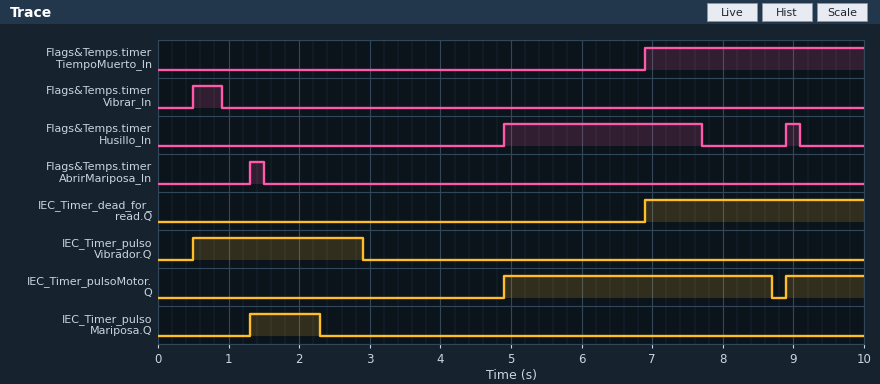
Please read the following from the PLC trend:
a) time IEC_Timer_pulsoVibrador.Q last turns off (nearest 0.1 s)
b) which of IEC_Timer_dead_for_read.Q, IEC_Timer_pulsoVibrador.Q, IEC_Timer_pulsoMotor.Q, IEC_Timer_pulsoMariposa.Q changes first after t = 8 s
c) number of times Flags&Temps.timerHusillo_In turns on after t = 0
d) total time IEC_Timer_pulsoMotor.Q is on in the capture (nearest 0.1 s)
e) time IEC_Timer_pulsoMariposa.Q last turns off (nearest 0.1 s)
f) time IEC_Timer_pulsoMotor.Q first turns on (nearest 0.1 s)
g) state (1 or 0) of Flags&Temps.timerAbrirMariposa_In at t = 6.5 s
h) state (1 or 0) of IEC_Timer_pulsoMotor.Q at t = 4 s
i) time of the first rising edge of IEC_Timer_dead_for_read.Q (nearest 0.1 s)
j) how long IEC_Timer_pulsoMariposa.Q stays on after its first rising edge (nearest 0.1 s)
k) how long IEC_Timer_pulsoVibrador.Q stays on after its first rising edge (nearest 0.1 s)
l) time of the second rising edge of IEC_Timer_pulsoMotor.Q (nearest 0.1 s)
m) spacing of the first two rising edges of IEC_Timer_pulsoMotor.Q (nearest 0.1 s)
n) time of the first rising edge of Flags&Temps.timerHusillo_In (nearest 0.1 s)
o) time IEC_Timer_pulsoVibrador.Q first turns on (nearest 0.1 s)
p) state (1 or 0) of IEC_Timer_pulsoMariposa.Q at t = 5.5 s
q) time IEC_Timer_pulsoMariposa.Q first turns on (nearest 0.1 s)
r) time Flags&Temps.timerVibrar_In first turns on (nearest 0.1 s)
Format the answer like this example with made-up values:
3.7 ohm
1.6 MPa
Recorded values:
2.9 s
IEC_Timer_pulsoMotor.Q
2
4.9 s
2.3 s
4.9 s
0
0
6.9 s
1.0 s
2.4 s
8.9 s
4.0 s
4.9 s
0.5 s
0
1.3 s
0.5 s
